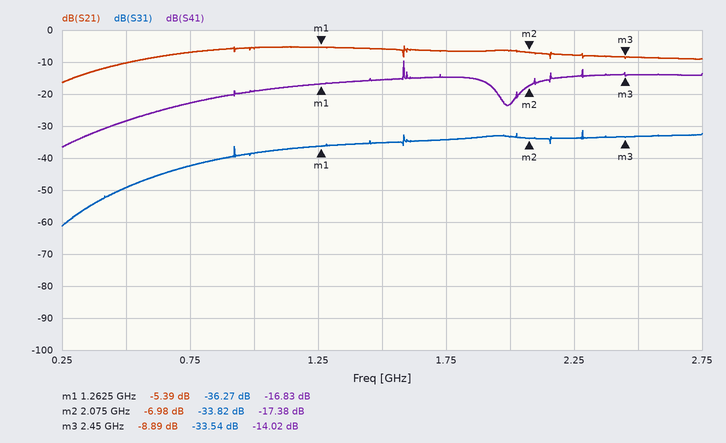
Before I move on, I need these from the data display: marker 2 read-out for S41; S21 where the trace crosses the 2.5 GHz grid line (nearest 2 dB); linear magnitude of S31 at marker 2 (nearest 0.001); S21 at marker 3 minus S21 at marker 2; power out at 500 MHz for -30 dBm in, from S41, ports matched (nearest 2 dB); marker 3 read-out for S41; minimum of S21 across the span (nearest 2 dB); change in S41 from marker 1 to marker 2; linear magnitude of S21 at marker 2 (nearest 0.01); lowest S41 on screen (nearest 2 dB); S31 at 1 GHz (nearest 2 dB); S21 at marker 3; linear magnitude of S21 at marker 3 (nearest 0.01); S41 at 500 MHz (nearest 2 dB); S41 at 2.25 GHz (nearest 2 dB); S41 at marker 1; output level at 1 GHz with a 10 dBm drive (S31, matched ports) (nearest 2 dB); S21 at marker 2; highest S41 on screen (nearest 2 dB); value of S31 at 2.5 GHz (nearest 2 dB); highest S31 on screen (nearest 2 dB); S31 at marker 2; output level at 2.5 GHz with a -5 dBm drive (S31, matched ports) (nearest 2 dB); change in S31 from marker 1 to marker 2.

-17.38 dB
-8 dB
0.020
-1.91 dB
-58 dBm
-14.02 dB
-16 dB
-0.55 dB
0.45
-36 dB
-38 dB
-8.89 dB
0.36
-28 dB
-14 dB
-16.83 dB
-28 dBm
-6.98 dB
-10 dB
-34 dB
-32 dB
-33.82 dB
-38 dBm
2.45 dB
